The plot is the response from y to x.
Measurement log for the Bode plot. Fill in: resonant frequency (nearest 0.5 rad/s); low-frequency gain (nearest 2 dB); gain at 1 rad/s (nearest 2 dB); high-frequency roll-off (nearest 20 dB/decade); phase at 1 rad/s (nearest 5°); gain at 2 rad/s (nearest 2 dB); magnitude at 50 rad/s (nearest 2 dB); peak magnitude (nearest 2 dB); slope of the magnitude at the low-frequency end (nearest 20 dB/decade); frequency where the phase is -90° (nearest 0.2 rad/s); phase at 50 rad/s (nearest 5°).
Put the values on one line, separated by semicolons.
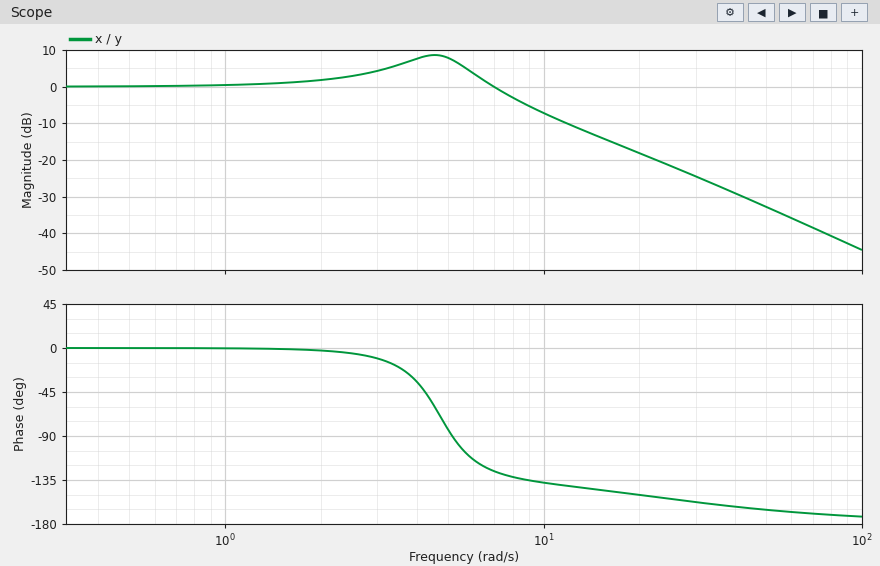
4.5 rad/s; 0 dB; 0 dB; -40 dB/decade; 0°; 2 dB; -32 dB; 8 dB; 0 dB/decade; 5.2 rad/s; -165°
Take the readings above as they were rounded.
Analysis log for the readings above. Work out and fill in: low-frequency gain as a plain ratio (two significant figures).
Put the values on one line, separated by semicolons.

1.0
